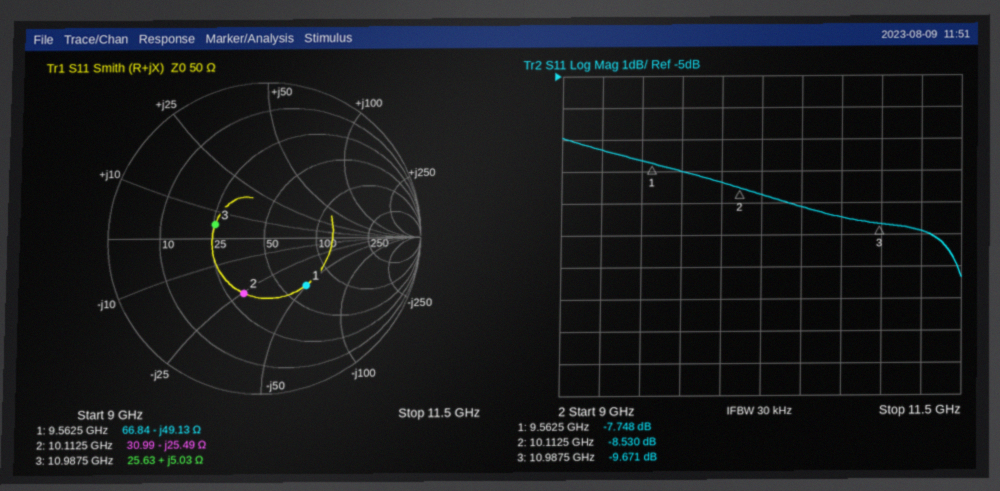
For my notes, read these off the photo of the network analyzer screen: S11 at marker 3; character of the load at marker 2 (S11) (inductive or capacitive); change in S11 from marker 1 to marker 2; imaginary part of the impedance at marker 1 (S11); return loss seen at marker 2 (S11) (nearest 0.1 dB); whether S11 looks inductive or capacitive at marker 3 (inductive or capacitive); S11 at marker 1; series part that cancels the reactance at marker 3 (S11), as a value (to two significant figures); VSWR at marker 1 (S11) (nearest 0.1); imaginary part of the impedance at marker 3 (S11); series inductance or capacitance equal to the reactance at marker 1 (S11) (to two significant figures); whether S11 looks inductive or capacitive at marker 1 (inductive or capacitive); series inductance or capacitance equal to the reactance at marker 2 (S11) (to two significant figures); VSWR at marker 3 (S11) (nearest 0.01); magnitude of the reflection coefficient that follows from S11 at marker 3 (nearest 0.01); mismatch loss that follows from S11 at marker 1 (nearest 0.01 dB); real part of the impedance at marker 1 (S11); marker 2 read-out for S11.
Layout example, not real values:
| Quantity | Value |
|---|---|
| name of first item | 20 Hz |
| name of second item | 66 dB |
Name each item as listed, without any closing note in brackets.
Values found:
| Quantity | Value |
|---|---|
| S11 at marker 3 | -9.671 dB |
| character of the load at marker 2 (S11) | capacitive |
| change in S11 from marker 1 to marker 2 | -0.782 dB |
| imaginary part of the impedance at marker 1 | -49.13 Ω |
| return loss seen at marker 2 (S11) | 8.5 dB |
| whether S11 looks inductive or capacitive at marker 3 | inductive |
| S11 at marker 1 | -7.748 dB |
| series part that cancels the reactance at marker 3 (S11), as a value | 2.9 pF |
| VSWR at marker 1 (S11) | 2.4 |
| imaginary part of the impedance at marker 3 | +5.03 Ω |
| series inductance or capacitance equal to the reactance at marker 1 (S11) | 340 fF |
| whether S11 looks inductive or capacitive at marker 1 | capacitive |
| series inductance or capacitance equal to the reactance at marker 2 (S11) | 620 fF |
| VSWR at marker 3 (S11) | 1.98 |
| magnitude of the reflection coefficient that follows from S11 at marker 3 | 0.33 |
| mismatch loss that follows from S11 at marker 1 | 0.80 dB |
| real part of the impedance at marker 1 | 66.84 Ω |
| marker 2 read-out for S11 | -8.530 dB |
